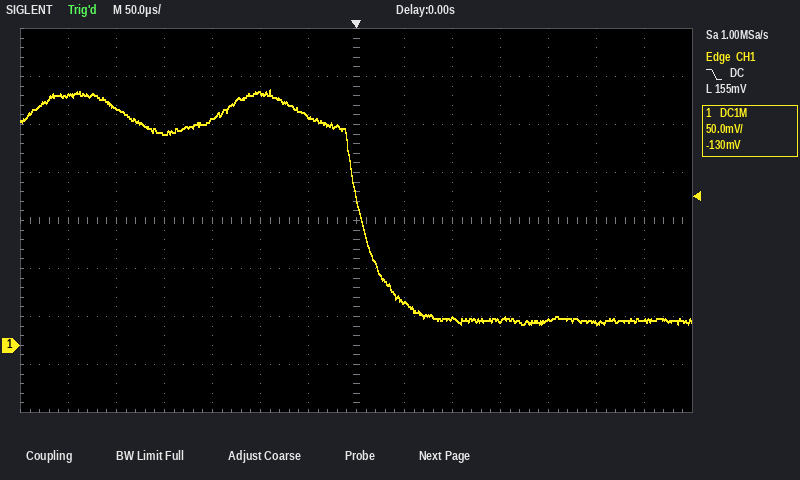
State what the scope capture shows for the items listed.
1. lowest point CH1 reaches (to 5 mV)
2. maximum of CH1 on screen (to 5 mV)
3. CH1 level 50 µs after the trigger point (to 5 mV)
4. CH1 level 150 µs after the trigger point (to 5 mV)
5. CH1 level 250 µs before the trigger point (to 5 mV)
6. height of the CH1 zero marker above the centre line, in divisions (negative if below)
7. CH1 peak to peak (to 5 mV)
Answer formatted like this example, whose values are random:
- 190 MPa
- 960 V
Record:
- 20 mV
- 265 mV
- 45 mV
- 25 mV
- 245 mV
- -2.6 div
- 245 mV
